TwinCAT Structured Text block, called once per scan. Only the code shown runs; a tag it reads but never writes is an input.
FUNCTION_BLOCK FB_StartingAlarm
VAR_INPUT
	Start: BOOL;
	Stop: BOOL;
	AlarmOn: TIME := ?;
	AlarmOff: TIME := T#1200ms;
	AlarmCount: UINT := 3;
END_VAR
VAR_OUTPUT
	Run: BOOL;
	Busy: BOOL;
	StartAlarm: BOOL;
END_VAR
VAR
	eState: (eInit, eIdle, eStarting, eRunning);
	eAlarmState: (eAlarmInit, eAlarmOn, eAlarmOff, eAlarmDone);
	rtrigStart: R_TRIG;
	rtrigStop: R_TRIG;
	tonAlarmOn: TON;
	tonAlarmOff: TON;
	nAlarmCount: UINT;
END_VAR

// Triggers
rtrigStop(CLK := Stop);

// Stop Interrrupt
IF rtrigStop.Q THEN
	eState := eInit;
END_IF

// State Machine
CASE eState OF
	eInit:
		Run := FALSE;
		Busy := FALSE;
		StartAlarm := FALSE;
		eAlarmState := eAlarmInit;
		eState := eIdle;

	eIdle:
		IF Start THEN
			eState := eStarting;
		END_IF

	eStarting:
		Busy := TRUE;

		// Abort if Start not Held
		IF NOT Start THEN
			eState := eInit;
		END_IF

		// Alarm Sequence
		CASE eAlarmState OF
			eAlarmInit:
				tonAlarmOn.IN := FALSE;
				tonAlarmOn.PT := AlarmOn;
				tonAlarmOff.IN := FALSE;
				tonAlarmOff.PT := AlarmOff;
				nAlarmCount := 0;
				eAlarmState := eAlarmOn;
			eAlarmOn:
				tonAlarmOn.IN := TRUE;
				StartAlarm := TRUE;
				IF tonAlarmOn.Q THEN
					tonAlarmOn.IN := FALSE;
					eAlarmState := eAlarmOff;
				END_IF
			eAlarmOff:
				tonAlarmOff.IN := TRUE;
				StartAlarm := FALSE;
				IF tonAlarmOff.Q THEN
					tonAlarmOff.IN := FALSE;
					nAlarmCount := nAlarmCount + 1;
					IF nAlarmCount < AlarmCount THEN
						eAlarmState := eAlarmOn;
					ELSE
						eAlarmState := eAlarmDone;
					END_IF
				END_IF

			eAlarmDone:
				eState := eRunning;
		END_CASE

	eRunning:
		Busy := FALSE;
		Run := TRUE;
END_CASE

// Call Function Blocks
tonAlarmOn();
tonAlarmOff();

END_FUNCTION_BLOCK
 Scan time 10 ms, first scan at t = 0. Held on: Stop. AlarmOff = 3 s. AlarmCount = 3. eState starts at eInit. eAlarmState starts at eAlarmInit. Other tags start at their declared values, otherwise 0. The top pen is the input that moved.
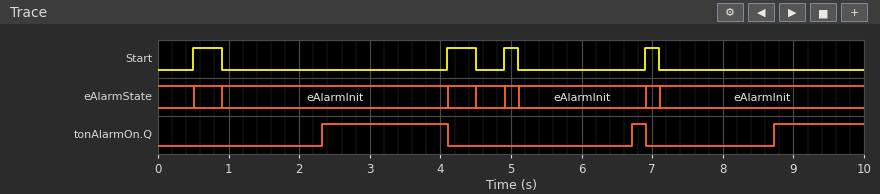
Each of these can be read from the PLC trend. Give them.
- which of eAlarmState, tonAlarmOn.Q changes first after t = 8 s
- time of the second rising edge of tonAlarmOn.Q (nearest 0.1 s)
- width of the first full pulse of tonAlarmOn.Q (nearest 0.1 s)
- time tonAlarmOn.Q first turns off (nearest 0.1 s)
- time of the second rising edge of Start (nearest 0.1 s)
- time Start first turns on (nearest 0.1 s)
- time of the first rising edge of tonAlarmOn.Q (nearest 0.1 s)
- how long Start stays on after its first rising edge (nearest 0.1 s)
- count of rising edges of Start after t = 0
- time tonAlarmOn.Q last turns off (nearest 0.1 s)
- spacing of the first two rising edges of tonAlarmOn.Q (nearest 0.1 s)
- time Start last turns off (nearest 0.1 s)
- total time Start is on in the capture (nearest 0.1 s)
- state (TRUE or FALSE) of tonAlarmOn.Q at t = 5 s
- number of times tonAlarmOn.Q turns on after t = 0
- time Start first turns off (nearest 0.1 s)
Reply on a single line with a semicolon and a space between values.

tonAlarmOn.Q; 6.7 s; 1.8 s; 4.1 s; 4.1 s; 0.5 s; 2.3 s; 0.4 s; 4; 6.9 s; 4.4 s; 7.1 s; 1.2 s; FALSE; 3; 0.9 s
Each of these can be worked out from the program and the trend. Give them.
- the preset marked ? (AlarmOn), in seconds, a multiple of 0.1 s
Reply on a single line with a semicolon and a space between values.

1.8 s
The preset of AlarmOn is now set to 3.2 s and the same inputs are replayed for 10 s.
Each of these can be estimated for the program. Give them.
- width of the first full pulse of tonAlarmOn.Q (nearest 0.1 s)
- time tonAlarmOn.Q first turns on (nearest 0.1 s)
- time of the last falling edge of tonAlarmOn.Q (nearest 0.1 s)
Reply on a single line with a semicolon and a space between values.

0.4 s; 3.7 s; 4.1 s
